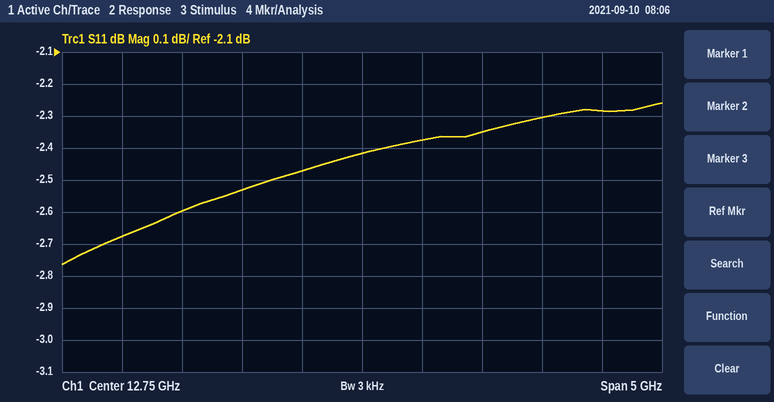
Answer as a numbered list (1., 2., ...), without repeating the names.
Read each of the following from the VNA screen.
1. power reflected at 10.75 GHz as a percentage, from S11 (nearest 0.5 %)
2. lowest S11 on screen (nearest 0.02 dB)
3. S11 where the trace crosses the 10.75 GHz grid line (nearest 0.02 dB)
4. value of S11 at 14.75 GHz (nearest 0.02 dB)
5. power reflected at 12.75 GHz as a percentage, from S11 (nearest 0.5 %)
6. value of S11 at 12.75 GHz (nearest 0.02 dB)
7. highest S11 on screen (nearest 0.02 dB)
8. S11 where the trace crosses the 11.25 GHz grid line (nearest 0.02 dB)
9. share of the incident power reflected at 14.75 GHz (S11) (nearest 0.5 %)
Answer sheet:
1. 54.0 %
2. -2.76 dB
3. -2.68 dB
4. -2.28 dB
5. 57.5 %
6. -2.42 dB
7. -2.26 dB
8. -2.60 dB
9. 59.0 %
